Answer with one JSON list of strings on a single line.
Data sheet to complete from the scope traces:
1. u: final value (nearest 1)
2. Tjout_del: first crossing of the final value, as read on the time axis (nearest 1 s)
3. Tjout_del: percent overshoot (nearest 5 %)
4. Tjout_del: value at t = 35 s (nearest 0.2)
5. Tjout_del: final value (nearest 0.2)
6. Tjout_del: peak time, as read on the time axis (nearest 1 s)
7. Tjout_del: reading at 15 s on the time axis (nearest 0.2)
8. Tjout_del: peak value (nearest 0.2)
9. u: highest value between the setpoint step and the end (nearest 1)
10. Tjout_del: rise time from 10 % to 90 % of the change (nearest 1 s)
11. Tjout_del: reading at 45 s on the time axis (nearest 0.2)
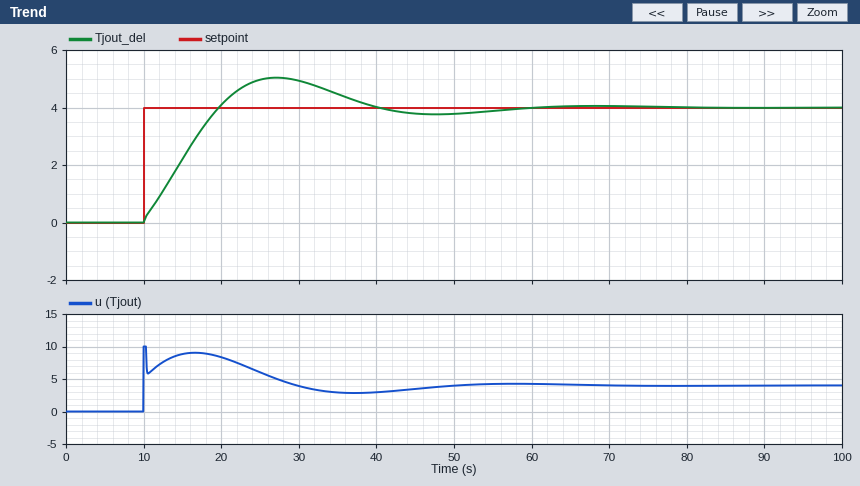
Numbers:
["4", "20 s", "25 %", "4.4", "4.0", "27 s", "2.2", "5.0", "10", "8 s", "3.8"]
